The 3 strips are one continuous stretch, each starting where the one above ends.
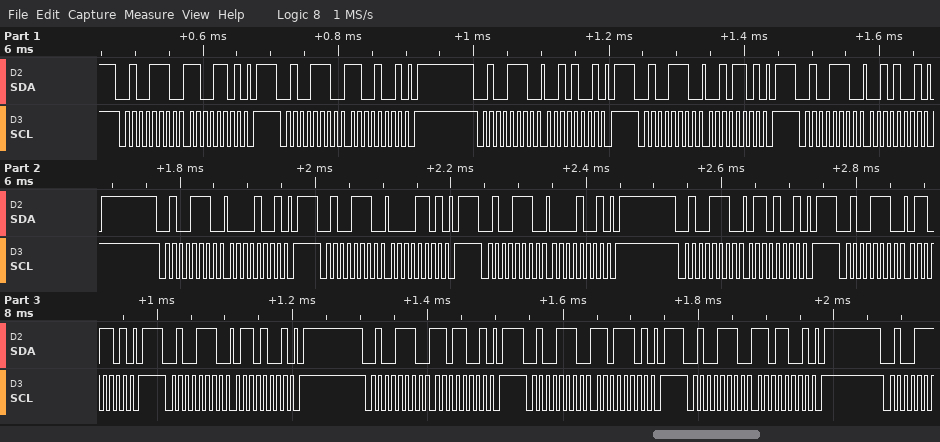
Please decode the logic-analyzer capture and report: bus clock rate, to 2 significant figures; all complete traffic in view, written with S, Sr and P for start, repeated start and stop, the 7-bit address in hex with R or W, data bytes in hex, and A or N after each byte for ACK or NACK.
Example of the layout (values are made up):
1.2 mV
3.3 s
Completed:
100 kHz
S 27W A CD A P S 27W A C9 A P S 27W A 29 A P S 27W A 2D A P S 27W A 29 A P S 27W A 09 A P S 27W A 0D A P S 27W A 09 A P S 27W A 69 A P S 27W A 6D A P S 27W A 69 A P S 27W A D9 A P S 27W A DD A P S 27W A D9 A P
